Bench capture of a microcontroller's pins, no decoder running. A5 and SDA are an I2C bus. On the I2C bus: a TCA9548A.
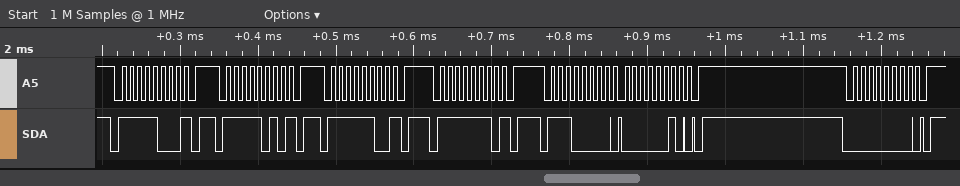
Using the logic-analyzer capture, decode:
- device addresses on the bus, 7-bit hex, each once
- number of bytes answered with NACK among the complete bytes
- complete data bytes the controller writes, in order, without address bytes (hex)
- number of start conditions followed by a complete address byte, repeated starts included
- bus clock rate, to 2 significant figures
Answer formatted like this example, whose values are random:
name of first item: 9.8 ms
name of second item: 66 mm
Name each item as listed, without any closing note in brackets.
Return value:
device addresses on the bus, 7-bit hex, each once: 0x7C 0x7D 0x7E 0x7F 0x70 0x00
number of bytes answered with NACK among the complete bytes: 4
complete data bytes the controller writes, in order, without address bytes: 02
number of start conditions followed by a complete address byte, repeated starts included: 6
bus clock rate, to 2 significant figures: 100 kHz
